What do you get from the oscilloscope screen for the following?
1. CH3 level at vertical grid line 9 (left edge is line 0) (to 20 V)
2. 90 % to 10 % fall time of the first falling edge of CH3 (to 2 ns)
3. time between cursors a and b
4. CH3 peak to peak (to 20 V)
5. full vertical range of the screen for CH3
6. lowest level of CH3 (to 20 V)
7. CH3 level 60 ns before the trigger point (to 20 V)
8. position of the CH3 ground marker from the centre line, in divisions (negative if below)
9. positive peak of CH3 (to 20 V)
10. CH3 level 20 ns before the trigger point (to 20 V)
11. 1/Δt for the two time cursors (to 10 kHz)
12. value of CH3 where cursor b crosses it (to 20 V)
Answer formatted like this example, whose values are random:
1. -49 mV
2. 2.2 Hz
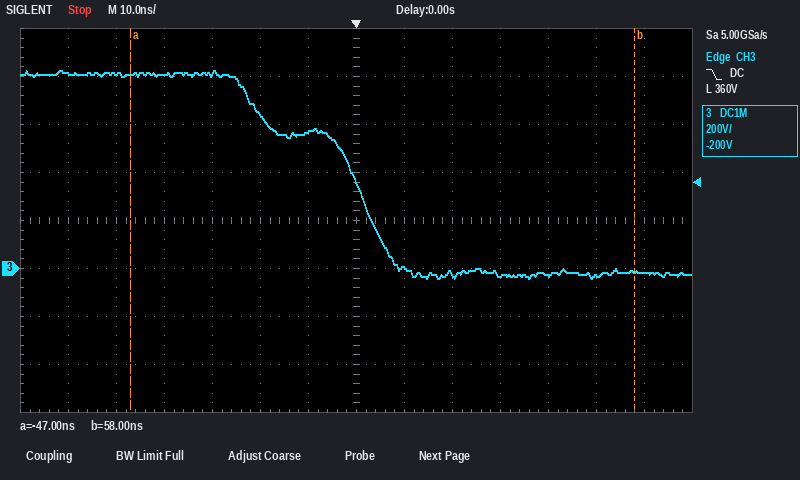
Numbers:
1. -20 V
2. 30 ns
3. 105 ns
4. 860 V
5. 1.6 kV
6. -40 V
7. 820 V
8. -1.0 div
9. 820 V
10. 640 V
11. 9.52 MHz
12. -20 V
